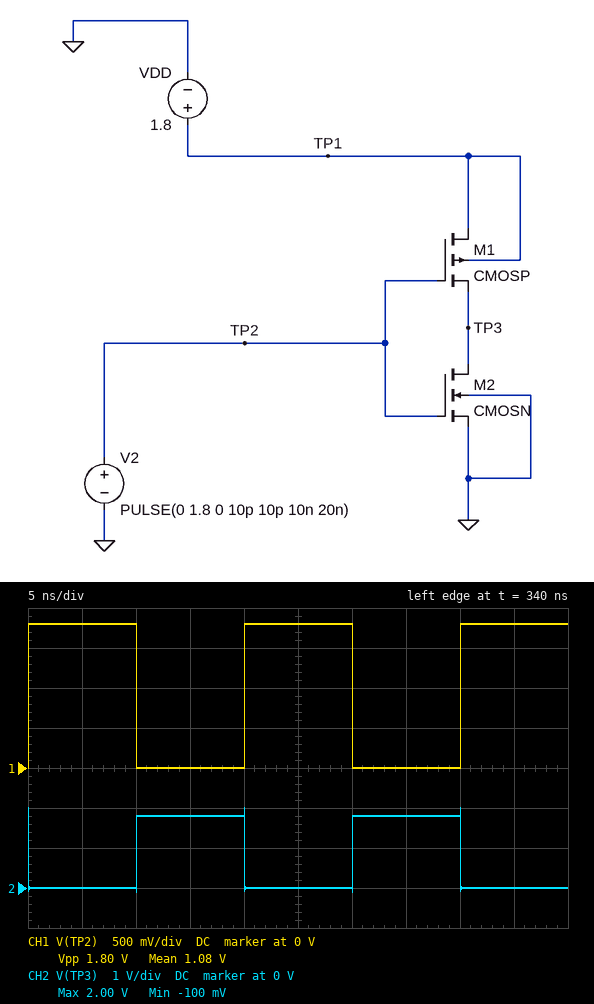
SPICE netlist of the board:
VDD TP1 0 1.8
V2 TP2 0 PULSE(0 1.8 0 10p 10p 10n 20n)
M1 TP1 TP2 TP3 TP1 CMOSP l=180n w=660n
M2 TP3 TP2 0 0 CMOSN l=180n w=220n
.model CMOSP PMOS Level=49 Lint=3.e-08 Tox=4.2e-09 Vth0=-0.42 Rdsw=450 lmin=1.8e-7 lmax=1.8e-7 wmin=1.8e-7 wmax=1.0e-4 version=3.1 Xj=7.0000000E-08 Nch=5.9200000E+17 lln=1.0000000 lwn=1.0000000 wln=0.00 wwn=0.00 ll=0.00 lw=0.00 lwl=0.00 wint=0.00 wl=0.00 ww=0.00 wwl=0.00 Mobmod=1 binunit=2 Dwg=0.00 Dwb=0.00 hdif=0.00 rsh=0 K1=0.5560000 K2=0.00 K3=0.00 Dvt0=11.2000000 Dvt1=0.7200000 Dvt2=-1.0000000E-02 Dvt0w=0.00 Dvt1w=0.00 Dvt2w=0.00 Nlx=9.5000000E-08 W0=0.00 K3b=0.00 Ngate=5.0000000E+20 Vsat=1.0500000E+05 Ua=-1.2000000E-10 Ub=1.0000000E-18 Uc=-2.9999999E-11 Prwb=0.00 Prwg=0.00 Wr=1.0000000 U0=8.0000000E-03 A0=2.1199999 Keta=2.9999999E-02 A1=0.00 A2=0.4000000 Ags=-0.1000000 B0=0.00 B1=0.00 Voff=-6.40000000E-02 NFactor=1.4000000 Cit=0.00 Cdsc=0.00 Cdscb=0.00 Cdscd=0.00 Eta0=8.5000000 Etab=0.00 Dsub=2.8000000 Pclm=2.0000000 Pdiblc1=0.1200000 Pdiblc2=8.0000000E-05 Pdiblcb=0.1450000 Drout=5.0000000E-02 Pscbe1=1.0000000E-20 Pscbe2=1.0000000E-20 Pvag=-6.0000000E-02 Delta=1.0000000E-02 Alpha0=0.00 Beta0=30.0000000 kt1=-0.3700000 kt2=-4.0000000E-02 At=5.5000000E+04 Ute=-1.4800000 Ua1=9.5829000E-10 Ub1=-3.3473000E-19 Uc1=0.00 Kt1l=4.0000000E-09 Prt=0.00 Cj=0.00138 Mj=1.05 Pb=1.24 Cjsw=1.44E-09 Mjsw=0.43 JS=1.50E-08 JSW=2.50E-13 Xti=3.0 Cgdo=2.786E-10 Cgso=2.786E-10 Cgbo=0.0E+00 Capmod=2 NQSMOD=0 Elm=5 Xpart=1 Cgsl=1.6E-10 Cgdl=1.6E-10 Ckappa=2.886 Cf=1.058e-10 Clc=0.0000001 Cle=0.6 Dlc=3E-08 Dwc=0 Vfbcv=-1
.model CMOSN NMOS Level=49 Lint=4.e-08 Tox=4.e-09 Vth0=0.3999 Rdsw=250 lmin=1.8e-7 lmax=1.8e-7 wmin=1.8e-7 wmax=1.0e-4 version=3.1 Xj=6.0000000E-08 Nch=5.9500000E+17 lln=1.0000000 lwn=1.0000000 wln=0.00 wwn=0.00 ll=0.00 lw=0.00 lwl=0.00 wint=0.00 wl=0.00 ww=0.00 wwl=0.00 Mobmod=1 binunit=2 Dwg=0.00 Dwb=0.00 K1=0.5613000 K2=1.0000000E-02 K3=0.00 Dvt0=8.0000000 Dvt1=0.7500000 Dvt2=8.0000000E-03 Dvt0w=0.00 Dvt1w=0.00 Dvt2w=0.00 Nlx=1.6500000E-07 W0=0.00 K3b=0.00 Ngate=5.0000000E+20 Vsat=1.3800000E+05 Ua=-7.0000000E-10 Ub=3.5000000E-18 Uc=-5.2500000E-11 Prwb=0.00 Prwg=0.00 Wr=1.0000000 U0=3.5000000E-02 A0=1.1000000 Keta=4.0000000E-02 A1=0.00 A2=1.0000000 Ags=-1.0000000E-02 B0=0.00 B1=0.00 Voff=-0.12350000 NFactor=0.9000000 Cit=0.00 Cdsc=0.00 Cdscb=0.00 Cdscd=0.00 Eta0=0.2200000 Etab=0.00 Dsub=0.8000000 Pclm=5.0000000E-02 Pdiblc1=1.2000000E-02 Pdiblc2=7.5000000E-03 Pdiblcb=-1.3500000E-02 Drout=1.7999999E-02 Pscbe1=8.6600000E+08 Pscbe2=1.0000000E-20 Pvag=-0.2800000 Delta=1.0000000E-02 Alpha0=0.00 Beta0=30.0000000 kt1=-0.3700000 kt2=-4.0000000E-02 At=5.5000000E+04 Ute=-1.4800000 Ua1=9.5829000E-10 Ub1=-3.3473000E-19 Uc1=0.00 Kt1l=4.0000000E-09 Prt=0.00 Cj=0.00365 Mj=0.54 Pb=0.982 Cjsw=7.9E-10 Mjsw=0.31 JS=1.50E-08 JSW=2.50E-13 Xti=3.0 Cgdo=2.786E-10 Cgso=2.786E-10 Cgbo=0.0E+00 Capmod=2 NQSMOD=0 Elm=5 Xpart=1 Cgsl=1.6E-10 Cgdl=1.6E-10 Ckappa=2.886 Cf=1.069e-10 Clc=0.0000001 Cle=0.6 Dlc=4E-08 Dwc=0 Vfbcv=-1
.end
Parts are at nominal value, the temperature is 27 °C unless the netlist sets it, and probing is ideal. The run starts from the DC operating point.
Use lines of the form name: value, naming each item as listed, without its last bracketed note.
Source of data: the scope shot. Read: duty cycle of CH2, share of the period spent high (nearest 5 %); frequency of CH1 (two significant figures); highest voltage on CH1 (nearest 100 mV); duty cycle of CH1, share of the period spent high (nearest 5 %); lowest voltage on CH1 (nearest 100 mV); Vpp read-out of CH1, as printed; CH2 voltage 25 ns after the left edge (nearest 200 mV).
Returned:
duty cycle of CH2, share of the period spent high: 50 %
frequency of CH1: 50 MHz
highest voltage on CH1: 1.8 V
duty cycle of CH1, share of the period spent high: 50 %
lowest voltage on CH1: 0 V
Vpp read-out of CH1, as printed: 1.80 V
CH2 voltage 25 ns after the left edge: 0 V
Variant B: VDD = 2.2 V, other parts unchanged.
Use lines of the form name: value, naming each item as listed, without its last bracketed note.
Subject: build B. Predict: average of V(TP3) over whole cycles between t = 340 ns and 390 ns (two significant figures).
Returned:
average of V(TP3) over whole cycles between t = 340 ns and 390 ns: 1.1 V
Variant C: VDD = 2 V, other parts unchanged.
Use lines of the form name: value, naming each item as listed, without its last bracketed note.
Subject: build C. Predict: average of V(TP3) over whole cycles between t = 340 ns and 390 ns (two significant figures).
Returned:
average of V(TP3) over whole cycles between t = 340 ns and 390 ns: 1.0 V
